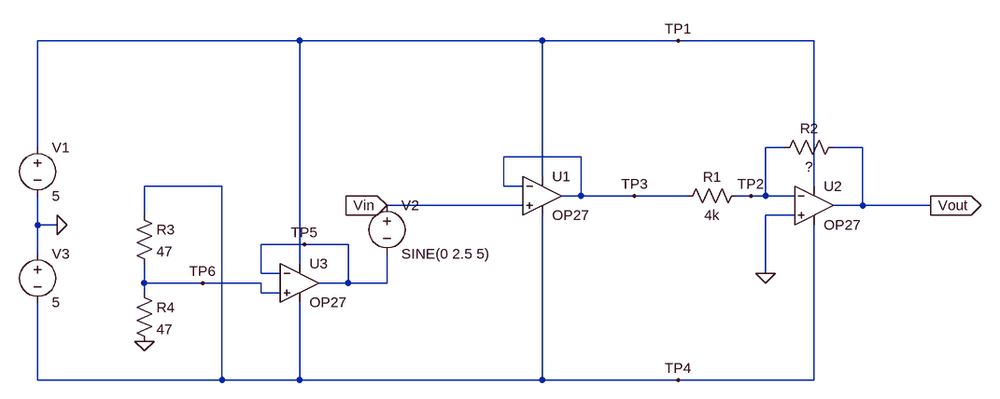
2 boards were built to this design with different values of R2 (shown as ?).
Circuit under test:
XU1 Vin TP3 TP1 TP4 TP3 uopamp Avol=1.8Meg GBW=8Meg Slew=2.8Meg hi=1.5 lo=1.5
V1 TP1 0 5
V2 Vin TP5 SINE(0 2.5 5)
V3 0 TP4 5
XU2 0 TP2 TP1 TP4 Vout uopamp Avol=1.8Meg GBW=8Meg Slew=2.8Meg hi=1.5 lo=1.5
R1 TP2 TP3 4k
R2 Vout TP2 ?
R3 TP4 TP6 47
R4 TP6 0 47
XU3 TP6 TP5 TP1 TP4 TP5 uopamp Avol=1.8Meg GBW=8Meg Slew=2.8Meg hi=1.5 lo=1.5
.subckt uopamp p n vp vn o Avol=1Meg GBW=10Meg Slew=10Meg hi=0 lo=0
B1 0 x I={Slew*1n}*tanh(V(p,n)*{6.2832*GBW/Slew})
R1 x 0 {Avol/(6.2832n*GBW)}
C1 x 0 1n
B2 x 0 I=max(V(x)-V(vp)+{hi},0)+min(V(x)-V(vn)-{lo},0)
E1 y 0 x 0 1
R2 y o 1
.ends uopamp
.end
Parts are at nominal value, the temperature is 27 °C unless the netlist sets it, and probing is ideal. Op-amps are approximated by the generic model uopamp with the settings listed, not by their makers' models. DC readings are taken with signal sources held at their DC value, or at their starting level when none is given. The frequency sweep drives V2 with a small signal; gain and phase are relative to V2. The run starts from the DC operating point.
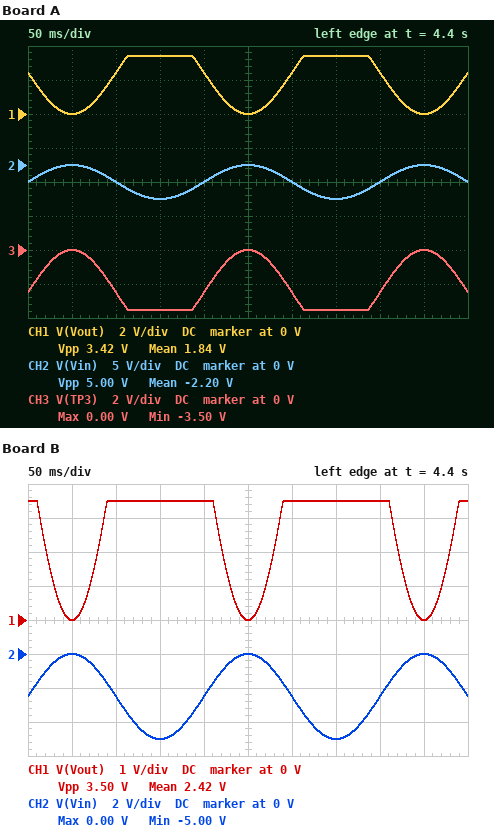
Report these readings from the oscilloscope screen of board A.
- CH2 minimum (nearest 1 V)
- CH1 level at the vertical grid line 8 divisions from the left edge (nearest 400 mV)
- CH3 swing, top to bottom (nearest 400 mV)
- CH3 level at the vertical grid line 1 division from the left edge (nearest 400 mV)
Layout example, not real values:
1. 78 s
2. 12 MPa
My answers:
1. -5 V
2. 2.4 V
3. 3.6 V
4. 0 V
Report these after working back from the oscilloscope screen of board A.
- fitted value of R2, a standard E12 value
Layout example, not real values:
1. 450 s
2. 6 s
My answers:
1. 3.9 kΩ
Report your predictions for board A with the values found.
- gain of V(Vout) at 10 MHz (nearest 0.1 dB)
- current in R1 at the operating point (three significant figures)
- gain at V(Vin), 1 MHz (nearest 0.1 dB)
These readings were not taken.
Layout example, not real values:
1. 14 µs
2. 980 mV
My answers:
1. -12.8 dB
2. 625 µA
3. 0 dB
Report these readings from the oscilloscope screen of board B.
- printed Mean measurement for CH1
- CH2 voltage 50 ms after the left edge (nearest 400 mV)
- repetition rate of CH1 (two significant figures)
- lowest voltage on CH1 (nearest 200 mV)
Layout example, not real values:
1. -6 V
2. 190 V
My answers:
1. 2.42 V
2. 0 V
3. 5.0 Hz
4. 0 V
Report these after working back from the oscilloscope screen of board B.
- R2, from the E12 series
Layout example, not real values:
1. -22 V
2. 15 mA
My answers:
1. 8.2 kΩ
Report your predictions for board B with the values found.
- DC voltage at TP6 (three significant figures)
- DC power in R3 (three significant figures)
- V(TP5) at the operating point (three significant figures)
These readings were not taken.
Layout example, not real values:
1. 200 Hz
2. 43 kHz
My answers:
1. -2.50 V
2. 133 mW
3. -2.50 V
